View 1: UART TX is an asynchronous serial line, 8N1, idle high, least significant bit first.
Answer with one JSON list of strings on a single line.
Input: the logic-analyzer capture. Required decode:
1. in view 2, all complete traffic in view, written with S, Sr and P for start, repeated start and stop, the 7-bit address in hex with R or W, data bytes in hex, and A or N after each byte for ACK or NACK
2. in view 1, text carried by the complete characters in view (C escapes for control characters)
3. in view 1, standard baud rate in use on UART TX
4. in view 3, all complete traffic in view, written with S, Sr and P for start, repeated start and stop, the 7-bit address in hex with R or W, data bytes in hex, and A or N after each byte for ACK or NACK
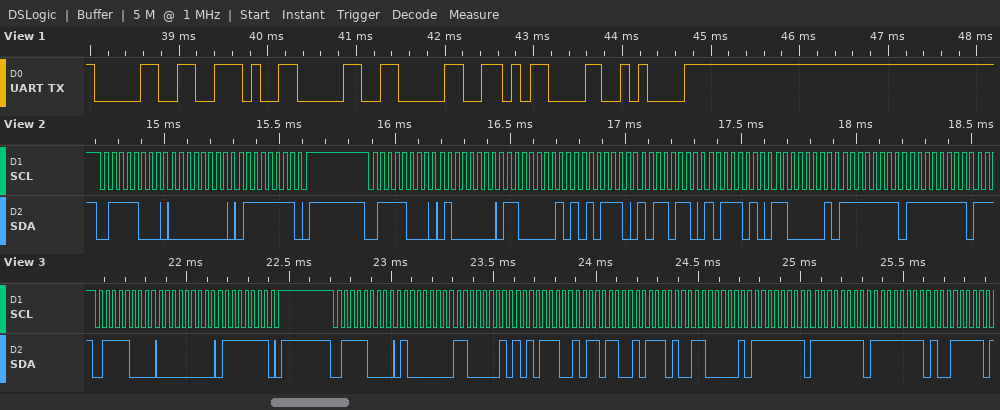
["S 3CW A 00 A 7F A P S 3CW A 40 A C1 A AE A B6 A BA A C1 A FF A FF A", "\"0.00\\r\\n\"", "9600 baud", "S 3CW A 00 A 7F A P S 3CW A 40 A C1 A AE A B6 A BA A C1 A FF A FF A FF A 9F A"]
